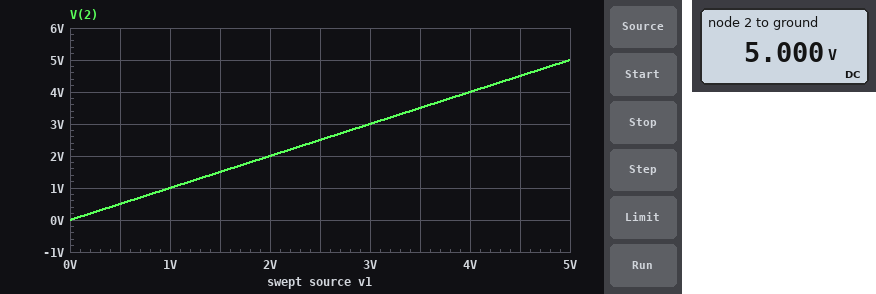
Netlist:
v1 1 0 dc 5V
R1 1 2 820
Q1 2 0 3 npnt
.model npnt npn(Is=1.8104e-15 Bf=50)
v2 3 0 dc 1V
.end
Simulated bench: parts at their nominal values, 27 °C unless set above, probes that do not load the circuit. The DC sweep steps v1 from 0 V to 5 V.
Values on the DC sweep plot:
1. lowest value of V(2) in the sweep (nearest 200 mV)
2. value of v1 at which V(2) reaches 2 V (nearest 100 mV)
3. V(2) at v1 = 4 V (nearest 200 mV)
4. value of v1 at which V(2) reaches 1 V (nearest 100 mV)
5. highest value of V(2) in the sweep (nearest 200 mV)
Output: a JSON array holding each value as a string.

["0 V", "2.0 V", "4.0 V", "1.0 V", "5.0 V"]
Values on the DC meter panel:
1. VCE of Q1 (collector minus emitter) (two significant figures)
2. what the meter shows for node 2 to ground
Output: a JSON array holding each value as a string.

["4.0 V", "5.000 V"]
